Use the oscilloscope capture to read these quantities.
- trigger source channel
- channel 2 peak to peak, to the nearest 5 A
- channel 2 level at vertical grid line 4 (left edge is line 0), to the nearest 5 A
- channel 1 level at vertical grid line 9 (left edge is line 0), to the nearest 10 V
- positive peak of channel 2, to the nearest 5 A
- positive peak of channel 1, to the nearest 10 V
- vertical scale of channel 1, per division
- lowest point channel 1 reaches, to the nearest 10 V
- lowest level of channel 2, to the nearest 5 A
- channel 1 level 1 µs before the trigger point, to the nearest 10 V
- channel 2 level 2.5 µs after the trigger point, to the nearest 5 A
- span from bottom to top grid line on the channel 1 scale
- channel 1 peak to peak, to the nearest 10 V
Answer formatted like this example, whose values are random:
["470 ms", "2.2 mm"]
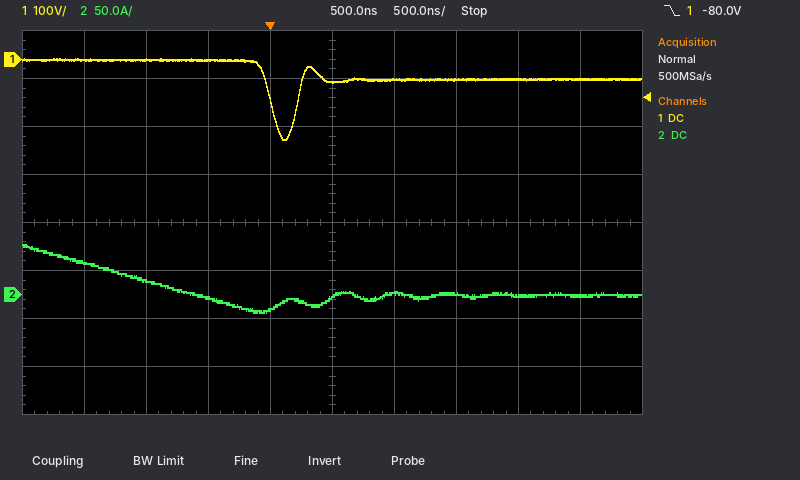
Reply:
["channel 1", "70 A", "-15 A", "-40 V", "50 A", "0 V", "100 V", "-170 V", "-20 A", "0 V", "0 A", "800 V", "170 V"]
